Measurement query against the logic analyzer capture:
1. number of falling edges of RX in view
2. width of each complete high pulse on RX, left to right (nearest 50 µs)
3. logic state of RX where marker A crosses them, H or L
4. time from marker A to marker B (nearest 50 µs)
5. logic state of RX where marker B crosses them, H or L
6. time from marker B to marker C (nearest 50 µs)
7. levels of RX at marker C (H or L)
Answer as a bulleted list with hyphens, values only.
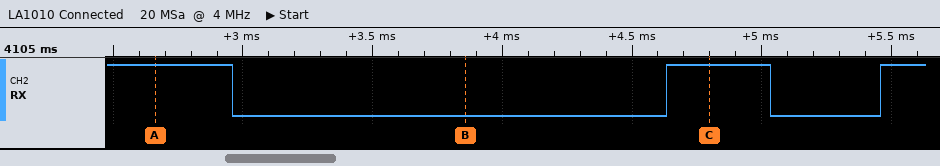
- 2
- 400 µs
- RX=H
- 1200 µs
- RX=L
- 950 µs
- RX=H
